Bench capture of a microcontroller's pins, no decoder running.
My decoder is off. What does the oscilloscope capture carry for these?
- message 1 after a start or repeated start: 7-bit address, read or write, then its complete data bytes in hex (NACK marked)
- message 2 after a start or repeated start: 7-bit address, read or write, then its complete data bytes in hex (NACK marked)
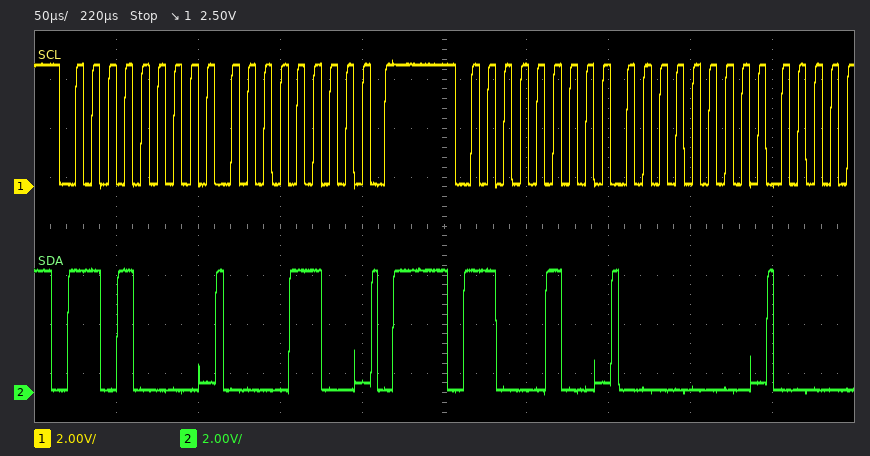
0x68 write: 0C
0x62 write: 00
